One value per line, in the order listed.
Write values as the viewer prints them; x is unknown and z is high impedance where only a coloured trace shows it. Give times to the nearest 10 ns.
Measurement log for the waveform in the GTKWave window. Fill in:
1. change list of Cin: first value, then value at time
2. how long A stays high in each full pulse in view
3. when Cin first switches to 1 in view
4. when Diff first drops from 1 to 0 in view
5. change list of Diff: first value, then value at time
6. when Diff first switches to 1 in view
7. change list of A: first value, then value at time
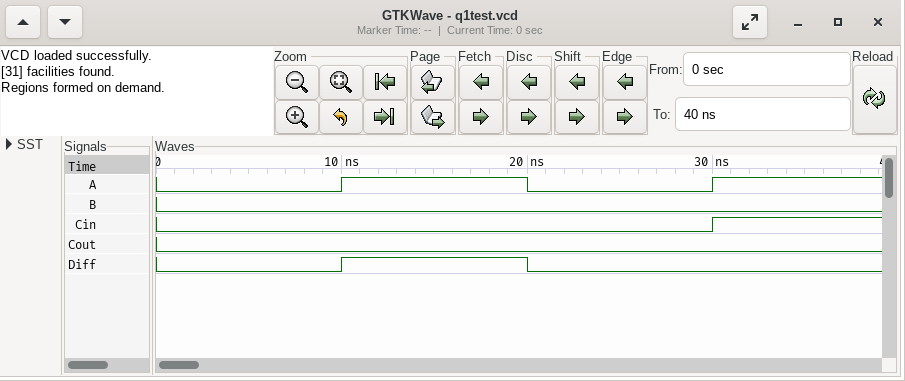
0, 1 at 30 ns
10 ns
30 ns
20 ns
0, 1 at 10 ns, 0 at 20 ns
10 ns
0, 1 at 10 ns, 0 at 20 ns, 1 at 30 ns
